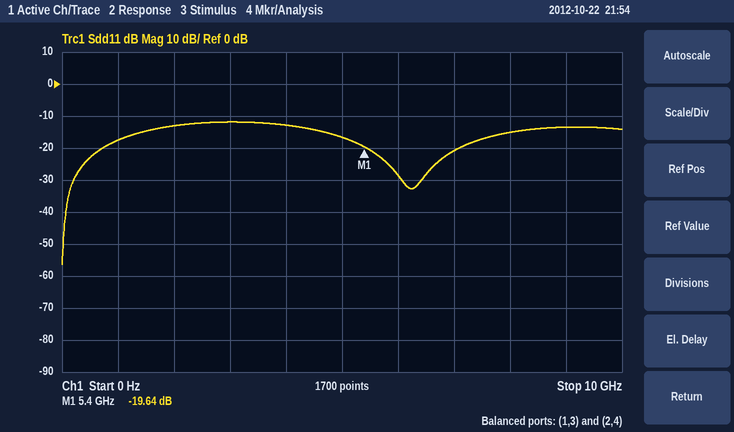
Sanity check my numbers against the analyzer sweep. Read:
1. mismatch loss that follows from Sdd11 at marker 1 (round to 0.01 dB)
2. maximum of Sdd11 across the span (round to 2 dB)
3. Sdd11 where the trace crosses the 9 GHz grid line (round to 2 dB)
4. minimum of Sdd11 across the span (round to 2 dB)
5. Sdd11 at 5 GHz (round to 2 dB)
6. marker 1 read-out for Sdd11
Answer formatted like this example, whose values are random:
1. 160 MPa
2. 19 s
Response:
1. 0.05 dB
2. -12 dB
3. -14 dB
4. -56 dB
5. -16 dB
6. -19.64 dB
